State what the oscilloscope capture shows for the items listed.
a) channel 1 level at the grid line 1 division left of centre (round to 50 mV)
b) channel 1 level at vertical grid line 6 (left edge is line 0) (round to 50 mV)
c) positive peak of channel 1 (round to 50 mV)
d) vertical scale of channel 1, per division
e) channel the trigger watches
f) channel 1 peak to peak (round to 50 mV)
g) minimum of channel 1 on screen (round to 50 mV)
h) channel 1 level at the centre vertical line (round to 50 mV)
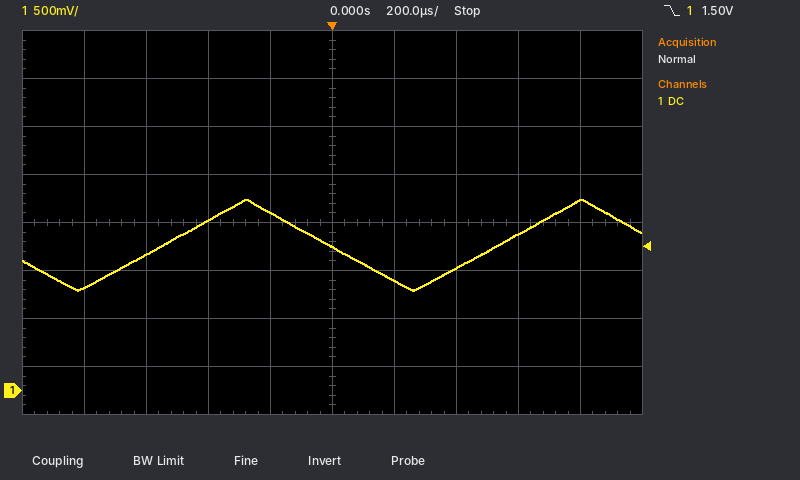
1.85 V
1.15 V
2.00 V
500 mV
channel 1
950 mV
1.05 V
1.50 V
